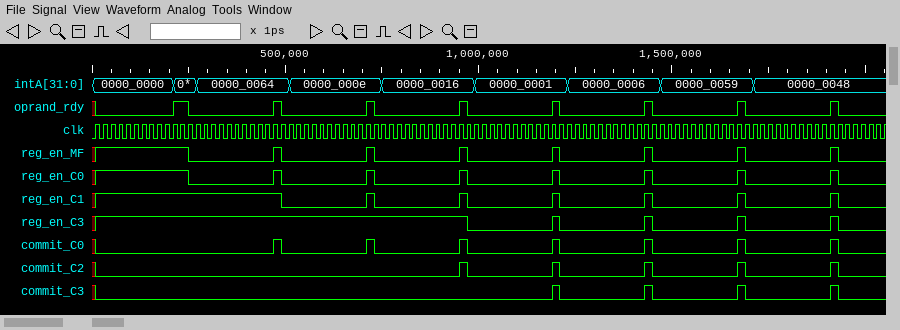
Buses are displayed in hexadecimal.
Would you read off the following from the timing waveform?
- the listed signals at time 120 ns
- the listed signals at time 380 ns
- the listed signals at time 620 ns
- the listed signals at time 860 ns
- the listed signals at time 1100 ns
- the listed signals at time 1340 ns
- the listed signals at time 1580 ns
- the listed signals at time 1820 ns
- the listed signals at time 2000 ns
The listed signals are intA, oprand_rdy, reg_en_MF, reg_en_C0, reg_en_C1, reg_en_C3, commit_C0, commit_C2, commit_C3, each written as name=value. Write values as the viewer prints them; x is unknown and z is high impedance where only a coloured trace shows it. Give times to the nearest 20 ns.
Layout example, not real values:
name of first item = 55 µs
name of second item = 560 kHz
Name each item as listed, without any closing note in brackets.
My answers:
the listed signals at time 120 ns = intA=0000_0000, oprand_rdy=0, reg_en_MF=1, reg_en_C0=1, reg_en_C1=1, reg_en_C3=1, commit_C0=0, commit_C2=0, commit_C3=0
the listed signals at time 380 ns = intA=0000_0064, oprand_rdy=0, reg_en_MF=0, reg_en_C0=0, reg_en_C1=1, reg_en_C3=1, commit_C0=0, commit_C2=0, commit_C3=0
the listed signals at time 620 ns = intA=0000_000e, oprand_rdy=0, reg_en_MF=0, reg_en_C0=0, reg_en_C1=0, reg_en_C3=1, commit_C0=0, commit_C2=0, commit_C3=0
the listed signals at time 860 ns = intA=0000_0016, oprand_rdy=0, reg_en_MF=0, reg_en_C0=0, reg_en_C1=0, reg_en_C3=1, commit_C0=0, commit_C2=0, commit_C3=0
the listed signals at time 1100 ns = intA=0000_0001, oprand_rdy=0, reg_en_MF=0, reg_en_C0=0, reg_en_C1=0, reg_en_C3=0, commit_C0=0, commit_C2=0, commit_C3=0
the listed signals at time 1340 ns = intA=0000_0006, oprand_rdy=0, reg_en_MF=0, reg_en_C0=0, reg_en_C1=0, reg_en_C3=0, commit_C0=0, commit_C2=0, commit_C3=0
the listed signals at time 1580 ns = intA=0000_0059, oprand_rdy=0, reg_en_MF=0, reg_en_C0=0, reg_en_C1=0, reg_en_C3=0, commit_C0=0, commit_C2=0, commit_C3=0
the listed signals at time 1820 ns = intA=0000_0048, oprand_rdy=0, reg_en_MF=0, reg_en_C0=0, reg_en_C1=0, reg_en_C3=0, commit_C0=0, commit_C2=0, commit_C3=0
the listed signals at time 2000 ns = intA=0000_0048, oprand_rdy=0, reg_en_MF=0, reg_en_C0=0, reg_en_C1=0, reg_en_C3=0, commit_C0=0, commit_C2=0, commit_C3=0
